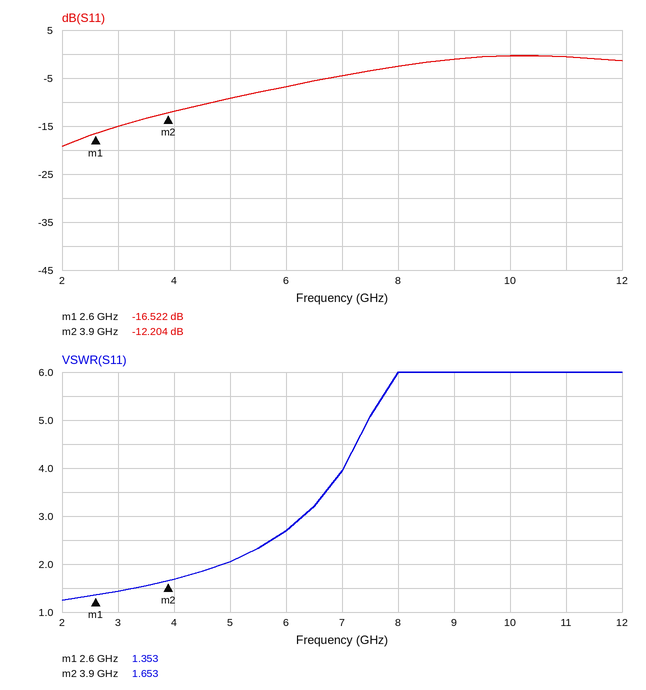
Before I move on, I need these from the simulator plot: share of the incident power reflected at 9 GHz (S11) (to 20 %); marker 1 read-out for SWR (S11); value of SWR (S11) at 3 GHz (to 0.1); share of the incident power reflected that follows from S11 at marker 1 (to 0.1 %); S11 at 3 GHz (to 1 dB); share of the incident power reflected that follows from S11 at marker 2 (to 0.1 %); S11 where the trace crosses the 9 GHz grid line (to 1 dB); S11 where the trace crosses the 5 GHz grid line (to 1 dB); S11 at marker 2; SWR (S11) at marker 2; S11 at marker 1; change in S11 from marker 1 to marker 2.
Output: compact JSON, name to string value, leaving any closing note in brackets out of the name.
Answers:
{"share of the incident power reflected at 9 GHz (S11)": "80 %", "marker 1 read-out for SWR": "1.353", "value of SWR (S11) at 3 GHz": "1.4", "share of the incident power reflected that follows from S11 at marker 1": "2.2 %", "S11 at 3 GHz": "-15 dB", "share of the incident power reflected that follows from S11 at marker 2": "6.0 %", "S11 where the trace crosses the 9 GHz grid line": "-1 dB", "S11 where the trace crosses the 5 GHz grid line": "-9 dB", "S11 at marker 2": "-12.204 dB", "SWR (S11) at marker 2": "1.653", "S11 at marker 1": "-16.522 dB", "change in S11 from marker 1 to marker 2": "4.318 dB"}
